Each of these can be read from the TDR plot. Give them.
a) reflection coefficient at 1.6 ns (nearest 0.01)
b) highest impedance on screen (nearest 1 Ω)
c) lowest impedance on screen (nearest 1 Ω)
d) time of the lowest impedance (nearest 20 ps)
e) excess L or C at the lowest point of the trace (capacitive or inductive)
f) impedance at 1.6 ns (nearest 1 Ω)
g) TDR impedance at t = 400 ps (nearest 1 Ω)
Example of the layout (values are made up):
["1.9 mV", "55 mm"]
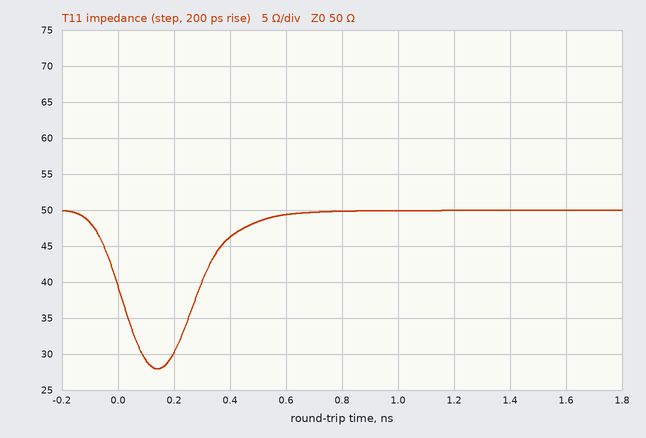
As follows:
["0.00", "50 Ω", "28 Ω", "140 ps", "capacitive", "50 Ω", "46 Ω"]
